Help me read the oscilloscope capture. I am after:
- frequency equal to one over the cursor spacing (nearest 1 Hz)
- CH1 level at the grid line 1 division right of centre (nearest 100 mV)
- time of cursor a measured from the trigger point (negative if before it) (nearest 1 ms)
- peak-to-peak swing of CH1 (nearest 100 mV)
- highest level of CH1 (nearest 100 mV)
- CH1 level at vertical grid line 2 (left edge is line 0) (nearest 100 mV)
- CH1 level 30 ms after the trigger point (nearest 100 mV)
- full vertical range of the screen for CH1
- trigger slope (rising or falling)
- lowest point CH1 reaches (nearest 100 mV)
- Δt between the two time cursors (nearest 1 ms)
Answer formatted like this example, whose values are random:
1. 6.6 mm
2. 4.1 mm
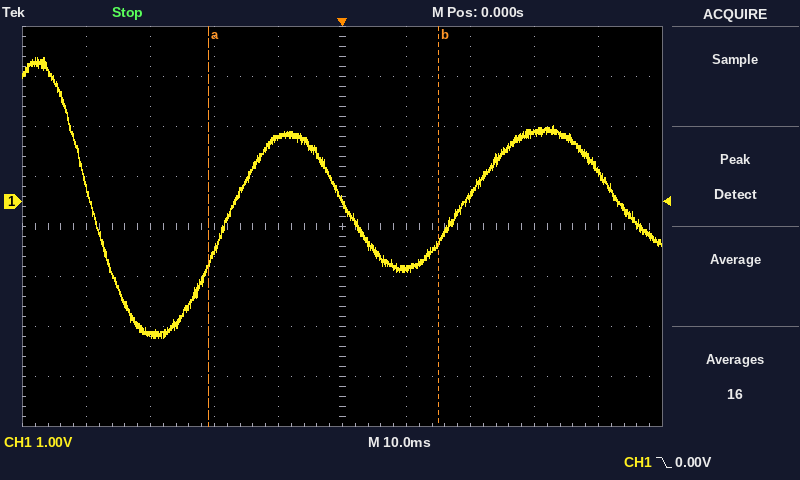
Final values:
1. 28 Hz
2. -1.3 V
3. -21 ms
4. 5.6 V
5. 2.9 V
6. -2.7 V
7. 1.4 V
8. 8 V
9. falling
10. -2.7 V
11. 36 ms
